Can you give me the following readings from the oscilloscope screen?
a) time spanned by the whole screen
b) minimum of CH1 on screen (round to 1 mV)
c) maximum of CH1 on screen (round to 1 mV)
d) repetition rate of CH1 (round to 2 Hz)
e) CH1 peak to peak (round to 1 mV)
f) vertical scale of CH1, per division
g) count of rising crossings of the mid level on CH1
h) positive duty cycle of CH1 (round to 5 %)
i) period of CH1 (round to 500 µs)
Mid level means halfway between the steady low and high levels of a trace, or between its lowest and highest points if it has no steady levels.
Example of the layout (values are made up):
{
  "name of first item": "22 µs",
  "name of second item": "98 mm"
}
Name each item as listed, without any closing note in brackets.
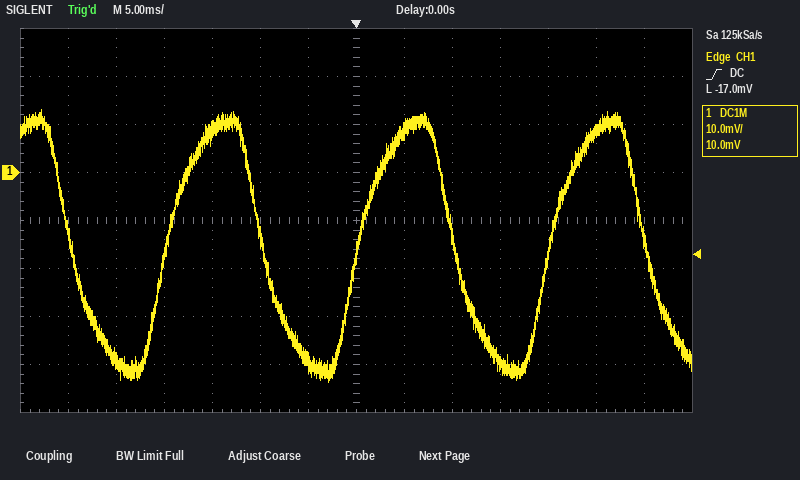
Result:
{
  "time spanned by the whole screen": "70 ms",
  "minimum of CH1 on screen": "-44 mV",
  "maximum of CH1 on screen": "13 mV",
  "repetition rate of CH1": "50 Hz",
  "CH1 peak to peak": "57 mV",
  "vertical scale of CH1, per division": "10 mV",
  "count of rising crossings of the mid level on CH1": "3",
  "positive duty cycle of CH1": "50 %",
  "period of CH1": "20.0 ms"
}
